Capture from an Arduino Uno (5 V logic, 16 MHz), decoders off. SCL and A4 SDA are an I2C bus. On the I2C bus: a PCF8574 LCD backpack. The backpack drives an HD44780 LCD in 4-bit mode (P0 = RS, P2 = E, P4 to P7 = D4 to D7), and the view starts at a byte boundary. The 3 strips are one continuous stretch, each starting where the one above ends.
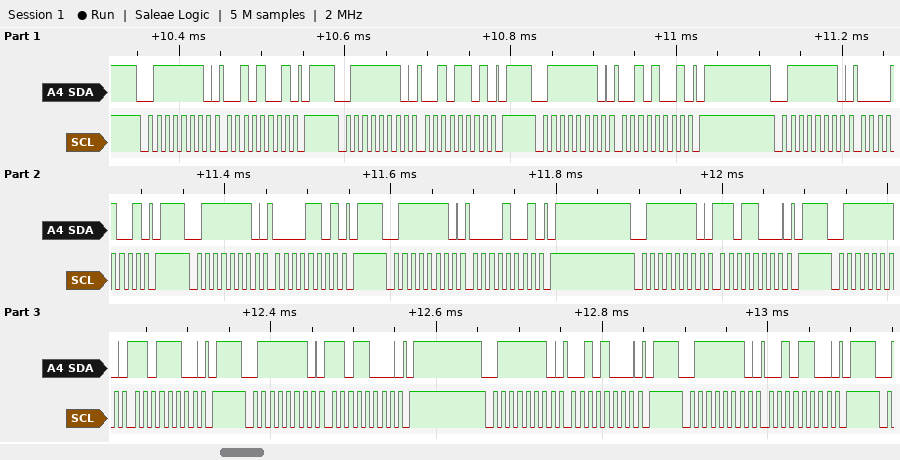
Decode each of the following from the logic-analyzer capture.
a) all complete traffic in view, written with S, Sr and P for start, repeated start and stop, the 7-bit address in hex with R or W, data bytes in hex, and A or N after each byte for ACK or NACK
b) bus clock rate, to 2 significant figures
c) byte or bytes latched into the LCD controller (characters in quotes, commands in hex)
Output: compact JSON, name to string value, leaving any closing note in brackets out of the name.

{"all complete traffic in view, written with S, Sr and P for start, repeated start and stop, the 7-bit address in hex with R or W, data bytes in hex, and A or N after each byte for ACK or NACK": "S 3FW A 29 A P S 3FW A 2D A P S 3FW A 29 A P S 3FW A 09 A P S 3FW A 0D A P S 3FW A 09 A P S 3FW A D8 A P S 3FW A DC A P S 3FW A D8 A P S 3FW A 28 A P S 3FW A 2C A P", "bus clock rate, to 2 significant figures": "100 kHz", "byte or bytes latched into the LCD controller": "' '"}
